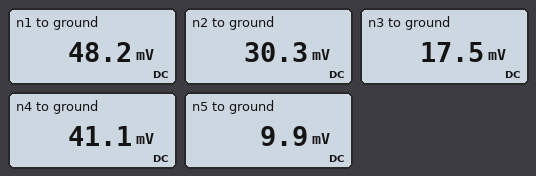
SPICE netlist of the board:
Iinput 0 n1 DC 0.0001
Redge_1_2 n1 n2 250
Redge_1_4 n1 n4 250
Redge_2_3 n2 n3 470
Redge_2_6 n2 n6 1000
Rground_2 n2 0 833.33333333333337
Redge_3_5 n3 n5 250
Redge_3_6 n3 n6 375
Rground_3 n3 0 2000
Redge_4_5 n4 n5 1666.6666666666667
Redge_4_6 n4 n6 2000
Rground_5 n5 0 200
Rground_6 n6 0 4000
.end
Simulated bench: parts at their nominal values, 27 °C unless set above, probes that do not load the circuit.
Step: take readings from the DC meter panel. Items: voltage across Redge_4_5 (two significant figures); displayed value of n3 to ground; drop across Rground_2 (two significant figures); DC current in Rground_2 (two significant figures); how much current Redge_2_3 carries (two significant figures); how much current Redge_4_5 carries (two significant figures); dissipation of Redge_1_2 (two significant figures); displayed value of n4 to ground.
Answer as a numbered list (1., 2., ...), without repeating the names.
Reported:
1. 31 mV
2. 17.5 mV
3. 30 mV
4. 36 µA
5. 27 µA
6. 19 µA
7. 1.3 µW
8. 41.1 mV
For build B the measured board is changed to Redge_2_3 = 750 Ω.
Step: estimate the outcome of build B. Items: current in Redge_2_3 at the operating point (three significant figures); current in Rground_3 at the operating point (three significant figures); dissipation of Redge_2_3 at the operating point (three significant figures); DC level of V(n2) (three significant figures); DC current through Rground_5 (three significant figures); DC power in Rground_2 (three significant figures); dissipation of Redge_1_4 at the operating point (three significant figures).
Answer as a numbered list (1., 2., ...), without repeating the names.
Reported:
1. 21.1 µA
2. 8.23 µA
3. 335 nW
4. 32.3 mV
5. 47.5 µA
6. 1.25 µW
7. 223 nW
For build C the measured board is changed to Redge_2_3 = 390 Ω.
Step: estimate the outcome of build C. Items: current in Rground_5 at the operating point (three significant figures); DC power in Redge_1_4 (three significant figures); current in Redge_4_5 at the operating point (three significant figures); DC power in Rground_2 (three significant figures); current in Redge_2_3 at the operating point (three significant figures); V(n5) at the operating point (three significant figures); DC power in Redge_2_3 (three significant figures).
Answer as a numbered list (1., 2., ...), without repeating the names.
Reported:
1. 50.1 µA
2. 191 nW
3. 18.4 µA
4. 1.04 µW
5. 29.6 µA
6. 10.0 mV
7. 341 nW
